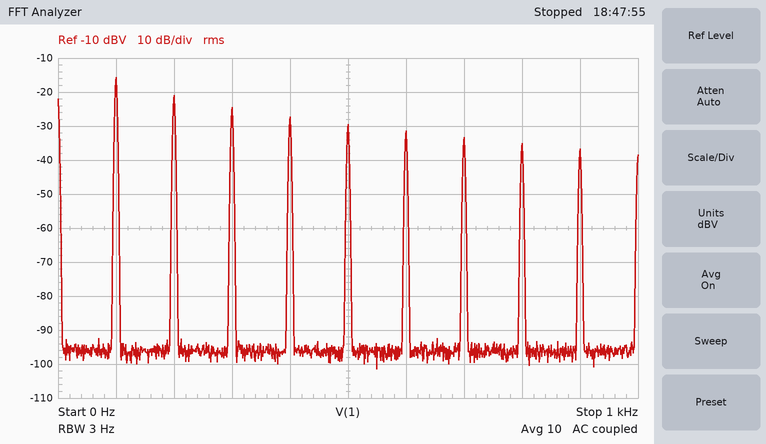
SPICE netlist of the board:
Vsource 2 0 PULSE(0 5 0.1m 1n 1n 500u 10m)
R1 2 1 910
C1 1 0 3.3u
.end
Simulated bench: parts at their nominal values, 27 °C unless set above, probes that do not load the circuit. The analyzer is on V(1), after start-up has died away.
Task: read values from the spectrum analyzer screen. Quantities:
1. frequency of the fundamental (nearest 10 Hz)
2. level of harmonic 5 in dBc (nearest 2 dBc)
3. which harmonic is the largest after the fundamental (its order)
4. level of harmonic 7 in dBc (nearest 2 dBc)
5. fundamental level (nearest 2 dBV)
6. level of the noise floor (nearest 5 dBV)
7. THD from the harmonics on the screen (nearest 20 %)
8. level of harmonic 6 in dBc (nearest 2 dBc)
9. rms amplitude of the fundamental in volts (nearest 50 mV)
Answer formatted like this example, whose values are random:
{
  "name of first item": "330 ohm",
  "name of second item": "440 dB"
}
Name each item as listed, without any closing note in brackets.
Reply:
{
  "frequency of the fundamental": "100 Hz",
  "level of harmonic 5 in dBc": "-14 dBc",
  "which harmonic is the largest after the fundamental": "2",
  "level of harmonic 7 in dBc": "-18 dBc",
  "fundamental level": "-16 dBV",
  "level of the noise floor": "-95 dBV",
  "THD from the harmonics on the screen": "80 %",
  "level of harmonic 6 in dBc": "-16 dBc",
  "rms amplitude of the fundamental in volts": "150 mV"
}
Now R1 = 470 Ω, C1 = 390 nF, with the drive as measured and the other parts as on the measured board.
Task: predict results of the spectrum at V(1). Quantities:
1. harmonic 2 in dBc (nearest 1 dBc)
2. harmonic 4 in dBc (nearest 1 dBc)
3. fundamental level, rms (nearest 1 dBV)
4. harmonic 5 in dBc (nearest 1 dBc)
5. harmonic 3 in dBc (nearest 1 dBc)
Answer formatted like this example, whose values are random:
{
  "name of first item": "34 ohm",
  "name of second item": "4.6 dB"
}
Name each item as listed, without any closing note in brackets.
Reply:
{
  "harmonic 2 in dBc": "0 dBc",
  "harmonic 4 in dBc": "-1 dBc",
  "fundamental level, rms": "-9 dBV",
  "harmonic 5 in dBc": "-2 dBc",
  "harmonic 3 in dBc": "-1 dBc"
}
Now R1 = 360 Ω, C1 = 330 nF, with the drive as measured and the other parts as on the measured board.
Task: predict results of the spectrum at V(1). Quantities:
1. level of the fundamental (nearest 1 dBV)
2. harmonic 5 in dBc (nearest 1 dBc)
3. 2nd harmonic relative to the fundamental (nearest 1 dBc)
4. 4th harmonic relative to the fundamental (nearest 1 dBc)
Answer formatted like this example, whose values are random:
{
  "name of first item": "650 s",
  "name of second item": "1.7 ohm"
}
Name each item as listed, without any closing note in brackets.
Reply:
{
  "level of the fundamental": "-9 dBV",
  "harmonic 5 in dBc": "-1 dBc",
  "2nd harmonic relative to the fundamental": "0 dBc",
  "4th harmonic relative to the fundamental": "-1 dBc"
}
